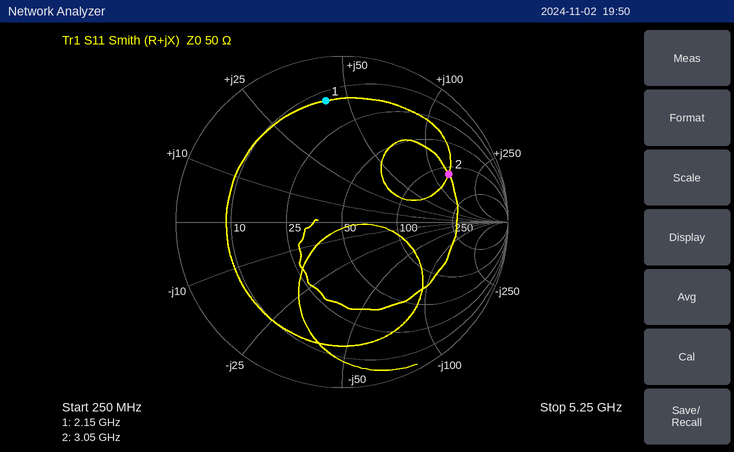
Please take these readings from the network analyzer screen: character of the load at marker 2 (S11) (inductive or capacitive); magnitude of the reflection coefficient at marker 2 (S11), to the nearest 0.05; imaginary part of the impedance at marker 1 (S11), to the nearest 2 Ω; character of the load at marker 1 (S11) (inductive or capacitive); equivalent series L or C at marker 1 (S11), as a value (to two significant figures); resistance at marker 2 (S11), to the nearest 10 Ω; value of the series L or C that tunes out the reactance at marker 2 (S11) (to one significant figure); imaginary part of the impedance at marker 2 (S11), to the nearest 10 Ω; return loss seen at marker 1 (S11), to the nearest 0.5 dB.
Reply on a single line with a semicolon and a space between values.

inductive; 0.70; +42 Ω; inductive; 3.1 nH; 120 Ω; 400 fF; +140 Ω; 2.5 dB
